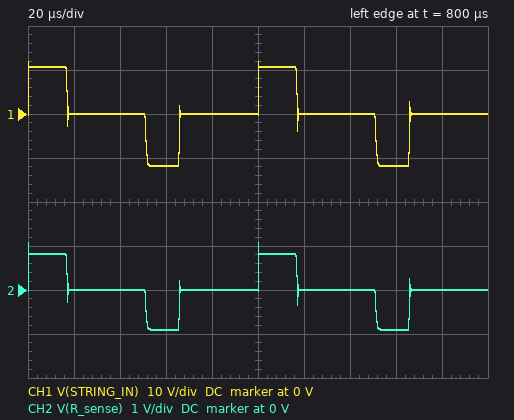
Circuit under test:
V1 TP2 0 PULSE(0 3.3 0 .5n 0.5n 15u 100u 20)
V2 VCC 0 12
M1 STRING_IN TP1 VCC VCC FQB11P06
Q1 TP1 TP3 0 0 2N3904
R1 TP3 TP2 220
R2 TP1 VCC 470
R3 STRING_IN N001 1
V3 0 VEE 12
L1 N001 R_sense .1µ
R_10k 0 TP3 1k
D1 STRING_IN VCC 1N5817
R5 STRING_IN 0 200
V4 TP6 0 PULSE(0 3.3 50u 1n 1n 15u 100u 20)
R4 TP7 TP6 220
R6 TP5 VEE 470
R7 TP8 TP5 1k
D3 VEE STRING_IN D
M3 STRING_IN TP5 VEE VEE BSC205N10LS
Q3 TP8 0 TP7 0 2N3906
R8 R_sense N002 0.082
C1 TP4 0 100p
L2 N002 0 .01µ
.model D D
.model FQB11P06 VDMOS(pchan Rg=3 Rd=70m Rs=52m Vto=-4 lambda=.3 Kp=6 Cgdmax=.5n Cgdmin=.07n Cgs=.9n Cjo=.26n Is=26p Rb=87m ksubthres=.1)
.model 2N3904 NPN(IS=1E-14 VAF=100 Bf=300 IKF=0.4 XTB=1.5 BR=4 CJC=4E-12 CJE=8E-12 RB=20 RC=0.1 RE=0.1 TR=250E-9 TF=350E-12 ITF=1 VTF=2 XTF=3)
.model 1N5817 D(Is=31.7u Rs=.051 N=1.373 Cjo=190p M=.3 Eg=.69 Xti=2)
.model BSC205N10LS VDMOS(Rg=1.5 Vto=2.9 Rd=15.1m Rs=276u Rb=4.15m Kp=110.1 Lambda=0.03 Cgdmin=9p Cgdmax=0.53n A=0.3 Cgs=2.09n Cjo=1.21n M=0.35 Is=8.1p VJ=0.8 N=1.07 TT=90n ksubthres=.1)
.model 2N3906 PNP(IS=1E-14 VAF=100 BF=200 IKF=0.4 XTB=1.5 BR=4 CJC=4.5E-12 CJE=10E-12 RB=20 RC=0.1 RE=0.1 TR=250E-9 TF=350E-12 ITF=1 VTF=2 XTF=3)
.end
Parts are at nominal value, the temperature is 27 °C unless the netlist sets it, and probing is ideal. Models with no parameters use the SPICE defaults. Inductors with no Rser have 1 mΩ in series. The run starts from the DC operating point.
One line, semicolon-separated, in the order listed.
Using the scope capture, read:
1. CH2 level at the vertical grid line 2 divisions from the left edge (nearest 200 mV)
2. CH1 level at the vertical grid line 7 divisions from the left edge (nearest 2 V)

0 V; 0 V
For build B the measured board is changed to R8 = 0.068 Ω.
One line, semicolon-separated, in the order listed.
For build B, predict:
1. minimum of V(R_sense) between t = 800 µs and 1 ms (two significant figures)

-760 mV
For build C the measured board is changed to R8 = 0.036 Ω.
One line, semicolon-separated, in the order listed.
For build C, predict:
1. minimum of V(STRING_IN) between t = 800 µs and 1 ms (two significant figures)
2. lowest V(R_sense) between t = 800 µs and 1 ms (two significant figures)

-12 V; -430 mV
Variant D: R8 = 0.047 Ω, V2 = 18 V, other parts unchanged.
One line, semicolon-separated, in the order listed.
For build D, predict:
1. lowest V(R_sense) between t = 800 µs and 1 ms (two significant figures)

-540 mV
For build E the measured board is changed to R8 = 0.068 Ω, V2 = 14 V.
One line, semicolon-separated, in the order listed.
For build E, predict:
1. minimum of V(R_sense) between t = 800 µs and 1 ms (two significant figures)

-760 mV
